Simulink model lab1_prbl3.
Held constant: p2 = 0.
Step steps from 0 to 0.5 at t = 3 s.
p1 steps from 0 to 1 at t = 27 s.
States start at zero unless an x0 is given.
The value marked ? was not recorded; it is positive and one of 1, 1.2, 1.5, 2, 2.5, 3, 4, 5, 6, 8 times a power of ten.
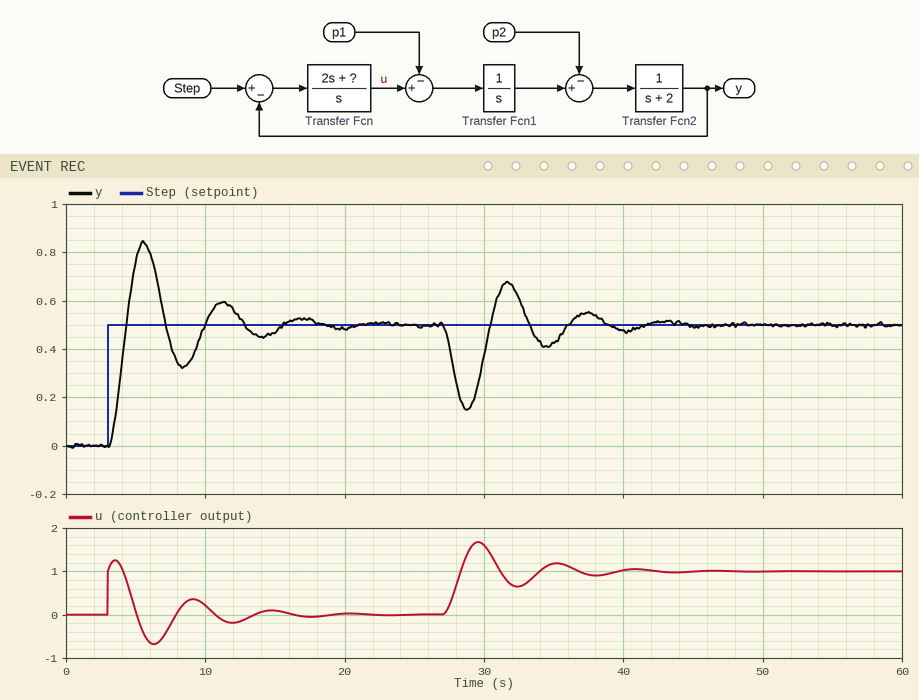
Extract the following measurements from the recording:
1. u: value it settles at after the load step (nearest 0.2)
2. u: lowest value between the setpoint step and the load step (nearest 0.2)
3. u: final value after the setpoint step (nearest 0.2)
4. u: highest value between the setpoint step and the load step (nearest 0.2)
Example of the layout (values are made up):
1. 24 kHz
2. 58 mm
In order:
1. 1.0
2. -0.6
3. 0.0
4. 1.2
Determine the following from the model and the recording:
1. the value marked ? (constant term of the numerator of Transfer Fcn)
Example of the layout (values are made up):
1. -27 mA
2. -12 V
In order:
1. 2
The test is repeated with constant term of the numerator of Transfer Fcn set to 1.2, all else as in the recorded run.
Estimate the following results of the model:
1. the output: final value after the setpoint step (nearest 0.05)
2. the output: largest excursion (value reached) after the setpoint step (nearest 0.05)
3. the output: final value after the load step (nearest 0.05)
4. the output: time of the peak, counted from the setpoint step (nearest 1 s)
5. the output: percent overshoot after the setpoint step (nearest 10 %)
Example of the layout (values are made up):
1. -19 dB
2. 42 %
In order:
1. 0.50
2. 0.75
3. 0.50
4. 3 s
5. 50 %
